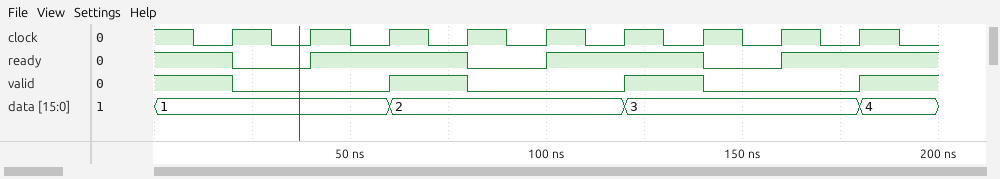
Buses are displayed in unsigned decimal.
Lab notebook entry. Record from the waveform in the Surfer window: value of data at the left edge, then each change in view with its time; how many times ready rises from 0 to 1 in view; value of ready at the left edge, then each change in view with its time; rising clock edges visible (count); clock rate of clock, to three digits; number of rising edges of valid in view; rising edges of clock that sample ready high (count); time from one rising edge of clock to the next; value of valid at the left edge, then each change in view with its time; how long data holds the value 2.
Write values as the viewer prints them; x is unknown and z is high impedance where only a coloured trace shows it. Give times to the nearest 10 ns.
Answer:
1, 2 at 60 ns, 3 at 120 ns, 4 at 180 ns
3
1, 0 at 20 ns, 1 at 40 ns, 0 at 80 ns, 1 at 100 ns, 0 at 140 ns, 1 at 160 ns
9
50.0 MHz
3
6
20 ns
1, 0 at 20 ns, 1 at 60 ns, 0 at 80 ns, 1 at 120 ns, 0 at 140 ns, 1 at 180 ns
60 ns
